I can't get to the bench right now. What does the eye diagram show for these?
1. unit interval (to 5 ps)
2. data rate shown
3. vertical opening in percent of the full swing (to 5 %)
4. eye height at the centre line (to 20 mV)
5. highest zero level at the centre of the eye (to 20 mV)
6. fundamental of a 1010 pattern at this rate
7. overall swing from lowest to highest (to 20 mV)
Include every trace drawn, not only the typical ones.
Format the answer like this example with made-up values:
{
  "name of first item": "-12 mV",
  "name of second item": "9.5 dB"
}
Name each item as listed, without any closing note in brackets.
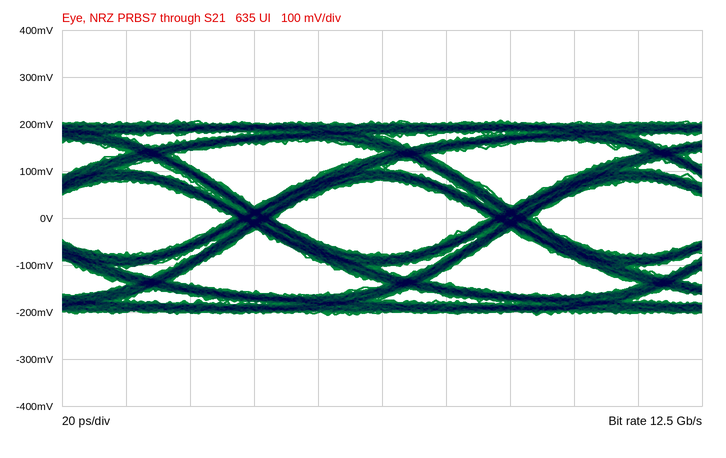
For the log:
{
  "unit interval": "80 ps",
  "data rate shown": "12.5 Gb/s",
  "vertical opening in percent of the full swing": "40 %",
  "eye height at the centre line": "160 mV",
  "highest zero level at the centre of the eye": "-80 mV",
  "fundamental of a 1010 pattern at this rate": "6.25 GHz",
  "overall swing from lowest to highest": "420 mV"
}
